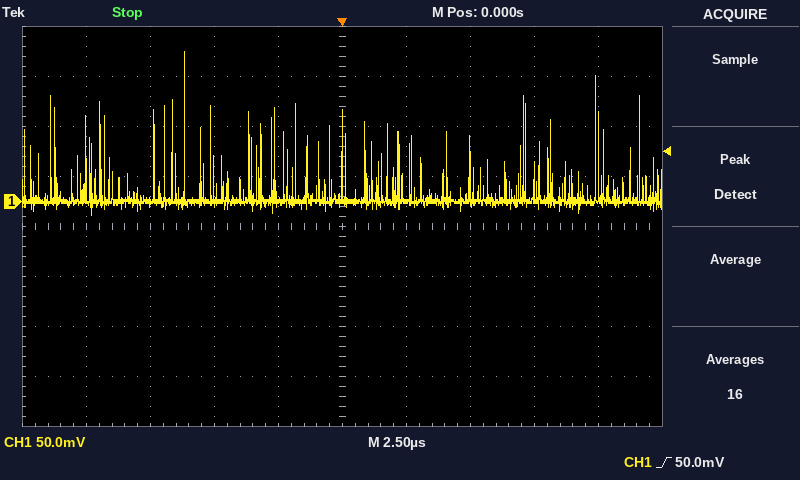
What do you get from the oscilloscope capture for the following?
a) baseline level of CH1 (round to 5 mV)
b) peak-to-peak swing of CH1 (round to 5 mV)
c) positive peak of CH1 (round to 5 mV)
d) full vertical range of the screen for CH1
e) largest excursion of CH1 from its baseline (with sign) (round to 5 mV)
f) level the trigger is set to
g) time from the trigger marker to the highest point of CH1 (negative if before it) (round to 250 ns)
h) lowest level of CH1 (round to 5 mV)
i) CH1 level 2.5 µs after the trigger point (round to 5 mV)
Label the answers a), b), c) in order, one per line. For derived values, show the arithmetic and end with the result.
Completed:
a) 0 mV
b) 150 mV − (-15 mV) = 165 mV
c) 150 mV
d) 400 mV
e) 150 mV − (0 mV) = +150 mV
f) 50.0 mV
g) -6.25 µs
h) -15 mV
i) 0 mV
